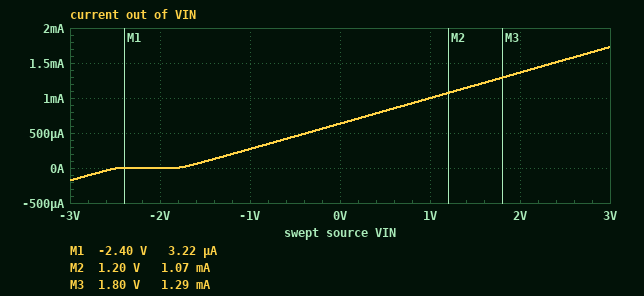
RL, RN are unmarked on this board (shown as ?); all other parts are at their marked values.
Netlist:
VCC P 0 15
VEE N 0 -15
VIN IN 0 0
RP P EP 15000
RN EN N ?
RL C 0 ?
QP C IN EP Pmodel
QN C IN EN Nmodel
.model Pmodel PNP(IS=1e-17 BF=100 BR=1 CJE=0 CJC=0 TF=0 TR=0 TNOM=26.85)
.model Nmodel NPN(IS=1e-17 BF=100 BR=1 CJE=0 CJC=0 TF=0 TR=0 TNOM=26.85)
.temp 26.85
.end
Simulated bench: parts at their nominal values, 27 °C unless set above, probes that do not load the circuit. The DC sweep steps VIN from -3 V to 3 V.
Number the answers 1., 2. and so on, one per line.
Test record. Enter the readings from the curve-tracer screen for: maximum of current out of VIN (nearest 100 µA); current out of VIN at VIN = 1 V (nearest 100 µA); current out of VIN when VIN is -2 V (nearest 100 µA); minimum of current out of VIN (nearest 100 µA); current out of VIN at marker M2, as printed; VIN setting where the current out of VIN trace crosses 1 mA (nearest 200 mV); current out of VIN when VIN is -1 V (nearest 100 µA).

1. 1.7 mA
2. 1.0 mA
3. 0 A
4. -200 µA
5. 1.07 mA
6. 1.0 V
7. 300 µA
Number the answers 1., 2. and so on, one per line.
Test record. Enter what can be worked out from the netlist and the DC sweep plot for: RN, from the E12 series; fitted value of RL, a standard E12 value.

1. 8.2 kΩ
2. 5.6 kΩ
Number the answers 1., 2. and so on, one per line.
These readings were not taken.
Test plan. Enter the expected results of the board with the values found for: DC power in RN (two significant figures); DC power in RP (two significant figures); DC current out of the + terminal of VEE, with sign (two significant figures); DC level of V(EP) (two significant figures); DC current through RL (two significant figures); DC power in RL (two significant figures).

1. 24 mW
2. 13 mW
3. -1.7 mA
4. 830 mV
5. 150 µA
6. 120 µW
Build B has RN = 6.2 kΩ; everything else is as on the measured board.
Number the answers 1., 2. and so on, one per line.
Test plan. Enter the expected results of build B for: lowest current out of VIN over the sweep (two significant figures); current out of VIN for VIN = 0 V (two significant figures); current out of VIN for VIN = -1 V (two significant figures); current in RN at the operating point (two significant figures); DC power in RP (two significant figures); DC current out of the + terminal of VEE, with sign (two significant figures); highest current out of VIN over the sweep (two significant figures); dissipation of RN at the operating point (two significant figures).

1. 6.8 µA
2. 1.2 mA
3. 780 µA
4. 2.3 mA
5. 13 mW
6. -2.3 mA
7. 2.4 mA
8. 32 mW
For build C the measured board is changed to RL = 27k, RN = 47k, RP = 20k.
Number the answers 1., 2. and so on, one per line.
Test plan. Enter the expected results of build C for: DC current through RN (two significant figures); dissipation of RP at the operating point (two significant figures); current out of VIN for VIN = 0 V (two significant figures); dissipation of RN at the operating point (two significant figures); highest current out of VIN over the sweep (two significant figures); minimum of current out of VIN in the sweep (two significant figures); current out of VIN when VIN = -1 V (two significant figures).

1. 300 µA
2. 10 mW
3. -380 µA
4. 4.3 mW
5. -54 µA
6. -700 µA
7. -480 µA
